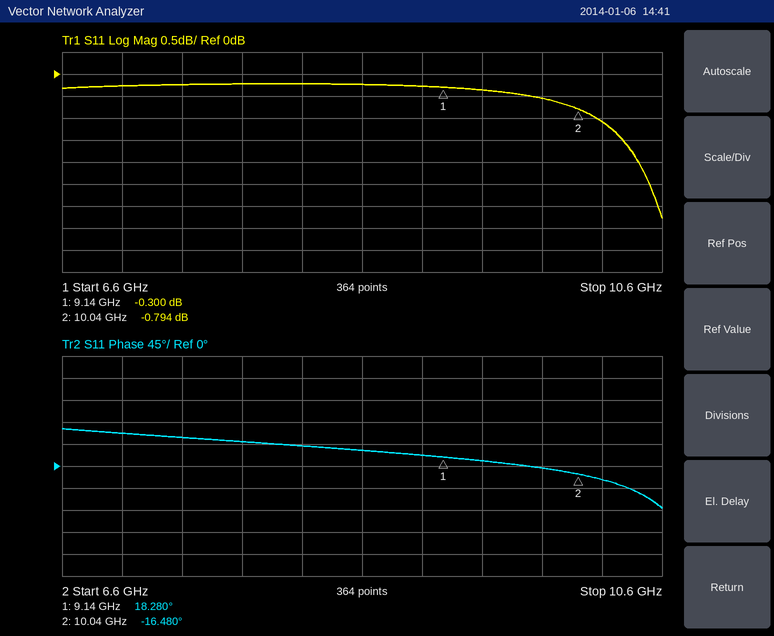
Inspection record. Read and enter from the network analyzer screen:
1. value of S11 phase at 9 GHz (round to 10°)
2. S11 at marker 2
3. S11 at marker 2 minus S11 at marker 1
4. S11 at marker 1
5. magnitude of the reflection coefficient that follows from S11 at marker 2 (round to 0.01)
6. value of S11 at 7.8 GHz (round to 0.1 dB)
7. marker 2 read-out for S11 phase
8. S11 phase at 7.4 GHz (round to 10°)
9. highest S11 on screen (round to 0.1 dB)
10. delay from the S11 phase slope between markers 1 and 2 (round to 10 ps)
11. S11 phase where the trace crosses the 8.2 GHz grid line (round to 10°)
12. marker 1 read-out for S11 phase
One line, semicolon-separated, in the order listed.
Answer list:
20°; -0.794 dB; -0.494 dB; -0.300 dB; 0.91; -0.2 dB; -16.480°; 60°; -0.2 dB; 110 ps; 40°; 18.280°
